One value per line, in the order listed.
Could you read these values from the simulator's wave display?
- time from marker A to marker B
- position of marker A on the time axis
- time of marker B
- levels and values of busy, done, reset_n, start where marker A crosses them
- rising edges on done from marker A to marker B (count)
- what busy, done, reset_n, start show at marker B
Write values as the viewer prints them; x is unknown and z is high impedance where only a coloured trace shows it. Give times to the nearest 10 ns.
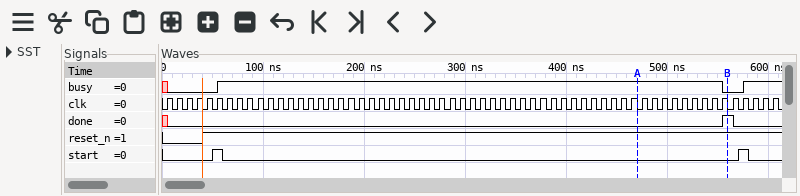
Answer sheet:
90 ns
470 ns
560 ns
busy=1, done=0, reset_n=1, start=0
1
busy=0, done=1, reset_n=1, start=0
